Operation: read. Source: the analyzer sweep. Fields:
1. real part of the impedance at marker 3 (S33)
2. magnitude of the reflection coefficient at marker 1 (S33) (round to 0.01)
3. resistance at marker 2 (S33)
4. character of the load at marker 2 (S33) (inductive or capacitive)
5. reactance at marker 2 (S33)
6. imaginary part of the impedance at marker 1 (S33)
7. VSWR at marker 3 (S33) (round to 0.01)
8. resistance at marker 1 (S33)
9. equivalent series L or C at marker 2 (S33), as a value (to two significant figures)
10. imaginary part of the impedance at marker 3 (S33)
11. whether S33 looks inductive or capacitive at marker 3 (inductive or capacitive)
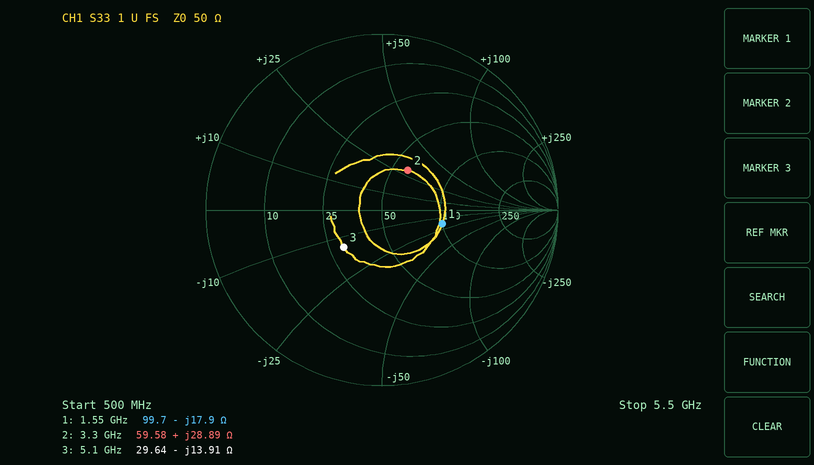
29.64 Ω
0.35
59.58 Ω
inductive
+28.89 Ω
-17.9 Ω
1.88
99.7 Ω
1.4 nH
-13.91 Ω
capacitive
